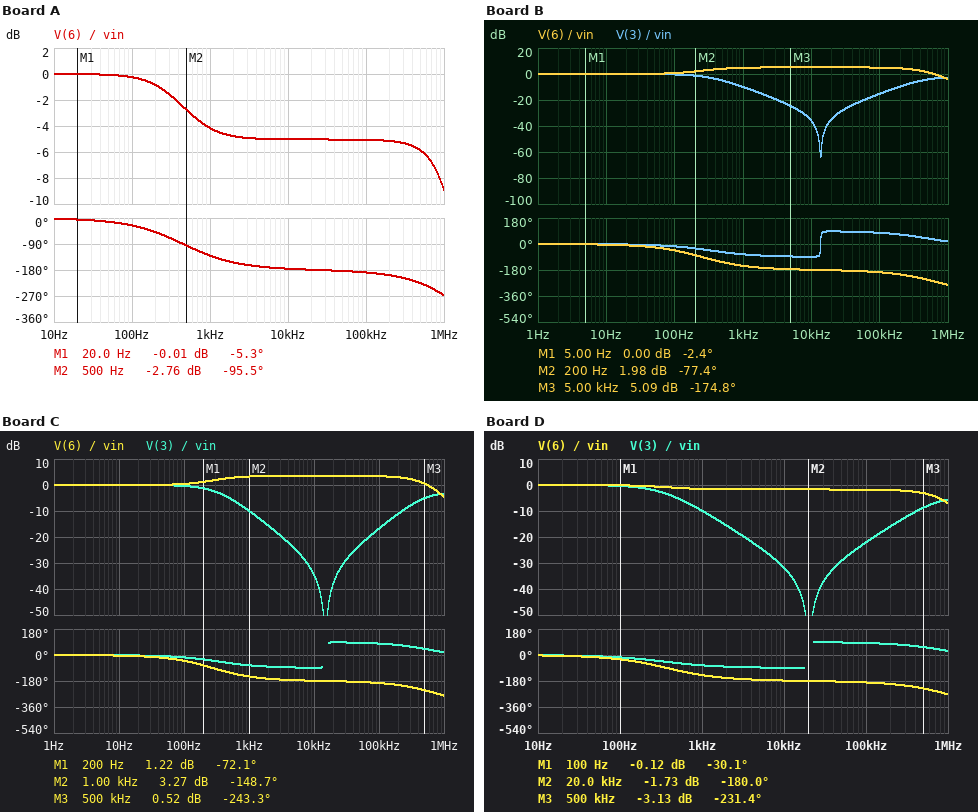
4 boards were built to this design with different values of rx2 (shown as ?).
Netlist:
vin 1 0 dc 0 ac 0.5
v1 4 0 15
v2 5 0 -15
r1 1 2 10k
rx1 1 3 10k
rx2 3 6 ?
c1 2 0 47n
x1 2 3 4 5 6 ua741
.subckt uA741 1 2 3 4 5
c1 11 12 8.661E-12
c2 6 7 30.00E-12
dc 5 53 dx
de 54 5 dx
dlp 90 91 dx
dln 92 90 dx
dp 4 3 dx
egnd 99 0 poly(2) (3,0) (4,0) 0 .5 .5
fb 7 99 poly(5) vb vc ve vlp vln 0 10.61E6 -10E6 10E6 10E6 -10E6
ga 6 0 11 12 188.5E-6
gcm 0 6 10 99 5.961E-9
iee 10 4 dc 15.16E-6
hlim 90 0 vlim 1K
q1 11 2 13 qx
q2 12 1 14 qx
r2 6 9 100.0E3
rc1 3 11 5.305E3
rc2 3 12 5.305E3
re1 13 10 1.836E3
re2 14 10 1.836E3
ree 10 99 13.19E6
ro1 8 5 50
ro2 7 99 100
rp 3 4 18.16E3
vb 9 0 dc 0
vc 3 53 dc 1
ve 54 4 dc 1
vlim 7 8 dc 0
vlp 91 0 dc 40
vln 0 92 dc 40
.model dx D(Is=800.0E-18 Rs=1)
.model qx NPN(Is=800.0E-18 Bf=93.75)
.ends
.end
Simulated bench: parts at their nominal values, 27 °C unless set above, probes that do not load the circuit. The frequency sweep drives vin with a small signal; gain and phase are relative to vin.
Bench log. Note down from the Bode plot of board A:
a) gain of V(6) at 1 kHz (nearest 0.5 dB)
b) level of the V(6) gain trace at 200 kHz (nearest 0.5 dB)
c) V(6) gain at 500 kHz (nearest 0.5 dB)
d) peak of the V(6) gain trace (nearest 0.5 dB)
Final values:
-4.0 dB
-5.0 dB
-6.0 dB
0 dB
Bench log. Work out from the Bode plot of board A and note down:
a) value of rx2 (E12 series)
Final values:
5.6 kΩ
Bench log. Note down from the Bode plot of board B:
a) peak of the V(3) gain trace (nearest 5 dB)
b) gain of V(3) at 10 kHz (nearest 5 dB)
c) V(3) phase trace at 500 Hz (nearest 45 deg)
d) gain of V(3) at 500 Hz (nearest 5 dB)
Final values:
0 dB
-35 dB
-45 deg
-5 dB
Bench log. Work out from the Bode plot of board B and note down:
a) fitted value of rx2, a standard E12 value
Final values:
18 kΩ
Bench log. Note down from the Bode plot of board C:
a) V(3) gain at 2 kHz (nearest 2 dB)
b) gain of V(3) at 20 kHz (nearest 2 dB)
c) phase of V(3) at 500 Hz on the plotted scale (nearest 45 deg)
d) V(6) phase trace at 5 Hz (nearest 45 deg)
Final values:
-16 dB
-38 dB
-45 deg
0 deg
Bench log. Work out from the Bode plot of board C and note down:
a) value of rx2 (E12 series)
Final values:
15 kΩ
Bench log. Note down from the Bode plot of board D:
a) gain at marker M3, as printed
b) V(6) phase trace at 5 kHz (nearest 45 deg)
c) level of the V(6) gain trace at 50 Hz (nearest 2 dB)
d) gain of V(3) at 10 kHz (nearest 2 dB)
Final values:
-3.13 dB
-180 deg
0 dB
-32 dB
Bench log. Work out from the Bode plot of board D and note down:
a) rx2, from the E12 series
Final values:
8.2 kΩ
